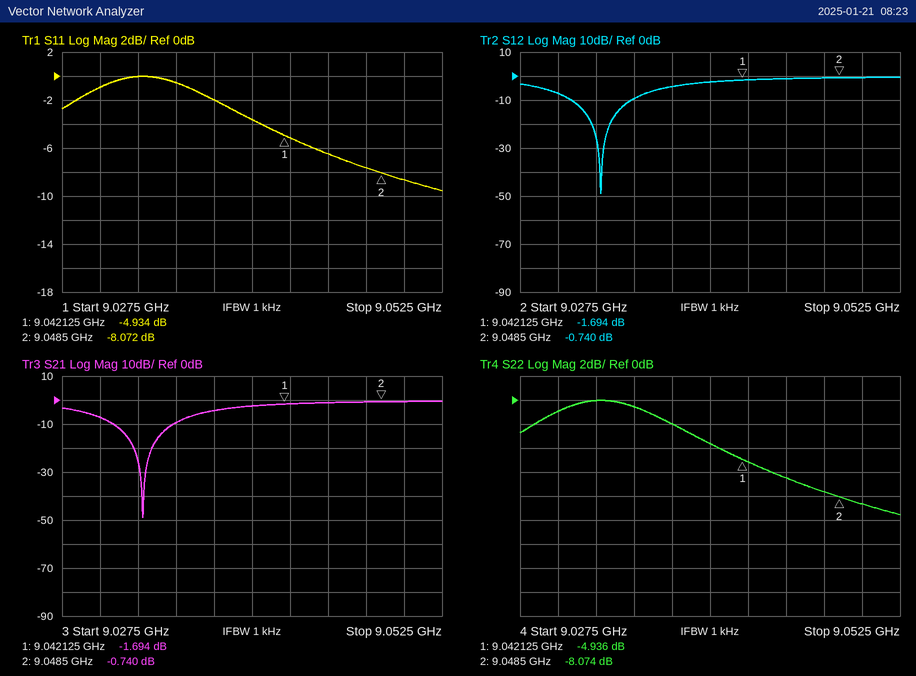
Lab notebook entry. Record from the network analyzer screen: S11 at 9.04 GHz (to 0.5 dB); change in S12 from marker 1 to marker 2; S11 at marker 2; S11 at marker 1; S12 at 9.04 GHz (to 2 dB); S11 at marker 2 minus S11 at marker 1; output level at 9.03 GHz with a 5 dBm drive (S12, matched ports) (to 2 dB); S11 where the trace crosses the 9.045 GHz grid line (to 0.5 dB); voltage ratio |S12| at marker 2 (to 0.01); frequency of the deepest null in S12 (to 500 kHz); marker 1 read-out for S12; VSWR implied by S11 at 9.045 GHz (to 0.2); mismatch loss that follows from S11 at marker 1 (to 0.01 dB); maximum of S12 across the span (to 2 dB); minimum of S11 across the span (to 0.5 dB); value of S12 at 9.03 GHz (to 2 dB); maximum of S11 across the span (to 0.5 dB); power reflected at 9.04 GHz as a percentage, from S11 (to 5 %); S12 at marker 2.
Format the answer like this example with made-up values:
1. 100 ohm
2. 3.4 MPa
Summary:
1. -3.5 dB
2. 0.954 dB
3. -8.072 dB
4. -4.934 dB
5. -2 dB
6. -3.138 dB
7. -2 dBm
8. -6.5 dB
9. 0.92
10. 9.0330 GHz
11. -1.694 dB
12. 2.8
13. 1.68 dB
14. 0 dB
15. -9.5 dB
16. -8 dB
17. 0.0 dB
18. 45 %
19. -0.740 dB
